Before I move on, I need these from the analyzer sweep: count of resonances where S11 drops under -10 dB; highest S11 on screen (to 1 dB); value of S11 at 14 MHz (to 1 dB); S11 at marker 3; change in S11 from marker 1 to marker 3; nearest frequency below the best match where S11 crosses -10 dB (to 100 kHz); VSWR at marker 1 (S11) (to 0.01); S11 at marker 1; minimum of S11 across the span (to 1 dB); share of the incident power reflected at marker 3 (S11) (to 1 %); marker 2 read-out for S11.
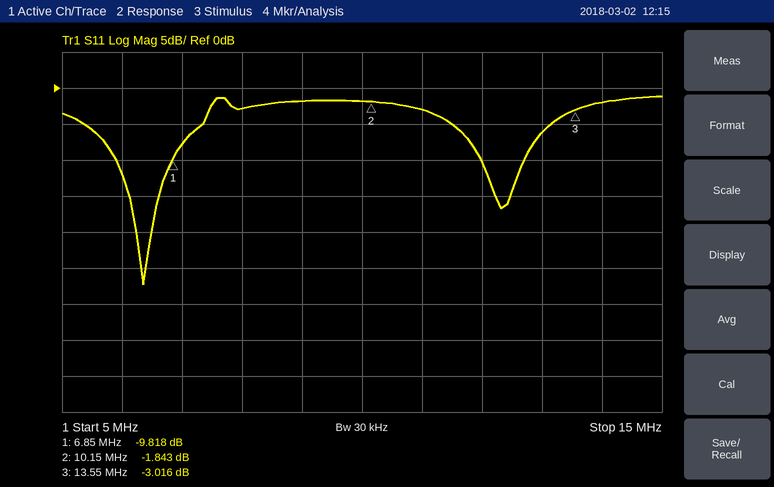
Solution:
2
-1 dB
-2 dB
-3.016 dB
6.802 dB
5.9 MHz
1.95
-9.818 dB
-27 dB
50 %
-1.843 dB
